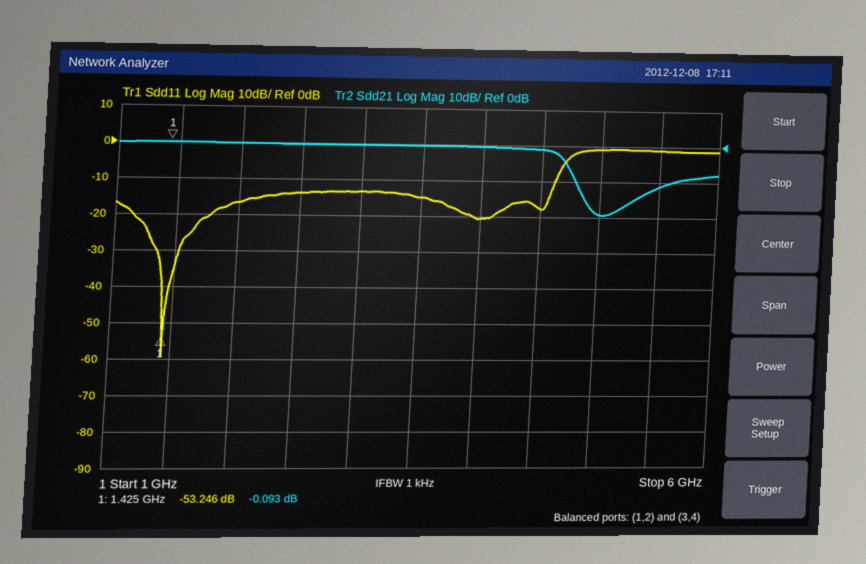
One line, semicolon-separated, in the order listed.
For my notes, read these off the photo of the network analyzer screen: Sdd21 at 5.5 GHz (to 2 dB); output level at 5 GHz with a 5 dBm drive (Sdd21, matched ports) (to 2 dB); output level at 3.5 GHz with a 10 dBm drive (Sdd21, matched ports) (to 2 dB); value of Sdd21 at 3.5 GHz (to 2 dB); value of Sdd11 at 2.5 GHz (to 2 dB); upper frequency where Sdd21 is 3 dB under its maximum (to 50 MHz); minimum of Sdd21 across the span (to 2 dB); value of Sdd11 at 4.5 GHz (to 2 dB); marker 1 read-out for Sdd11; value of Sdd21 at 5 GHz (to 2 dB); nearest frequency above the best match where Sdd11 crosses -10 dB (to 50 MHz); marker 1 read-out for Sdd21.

-12 dB; -14 dBm; 10 dBm; 0 dB; -14 dB; 4.65 GHz; -20 dB; -18 dB; -53.246 dB; -20 dB; 4.60 GHz; -0.093 dB
